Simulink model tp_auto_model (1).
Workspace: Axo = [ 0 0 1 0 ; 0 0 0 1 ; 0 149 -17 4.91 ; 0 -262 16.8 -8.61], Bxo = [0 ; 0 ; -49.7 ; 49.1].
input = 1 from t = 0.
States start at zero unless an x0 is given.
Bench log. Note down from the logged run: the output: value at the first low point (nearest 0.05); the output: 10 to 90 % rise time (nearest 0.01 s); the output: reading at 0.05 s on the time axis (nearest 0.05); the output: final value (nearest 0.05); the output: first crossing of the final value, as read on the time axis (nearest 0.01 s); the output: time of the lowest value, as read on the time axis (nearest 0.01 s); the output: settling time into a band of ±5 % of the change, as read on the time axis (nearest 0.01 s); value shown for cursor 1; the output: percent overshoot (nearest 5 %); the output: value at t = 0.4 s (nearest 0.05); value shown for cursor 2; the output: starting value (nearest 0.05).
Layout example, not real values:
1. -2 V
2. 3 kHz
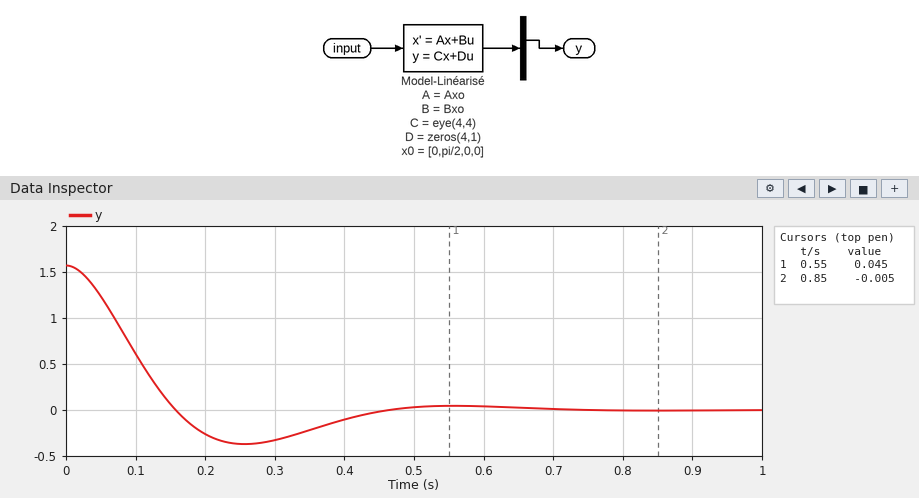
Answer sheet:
1. -0.35
2. 0.11 s
3. 1.25
4. 0.00
5. 0.16 s
6. 0.26 s
7. 0.41 s
8. 0.045
9. 25 %
10. -0.10
11. -0.005
12. 1.55
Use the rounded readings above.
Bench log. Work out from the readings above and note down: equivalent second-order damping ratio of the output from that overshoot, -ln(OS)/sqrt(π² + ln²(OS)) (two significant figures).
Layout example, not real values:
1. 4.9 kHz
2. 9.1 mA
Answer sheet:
1. 0.40
